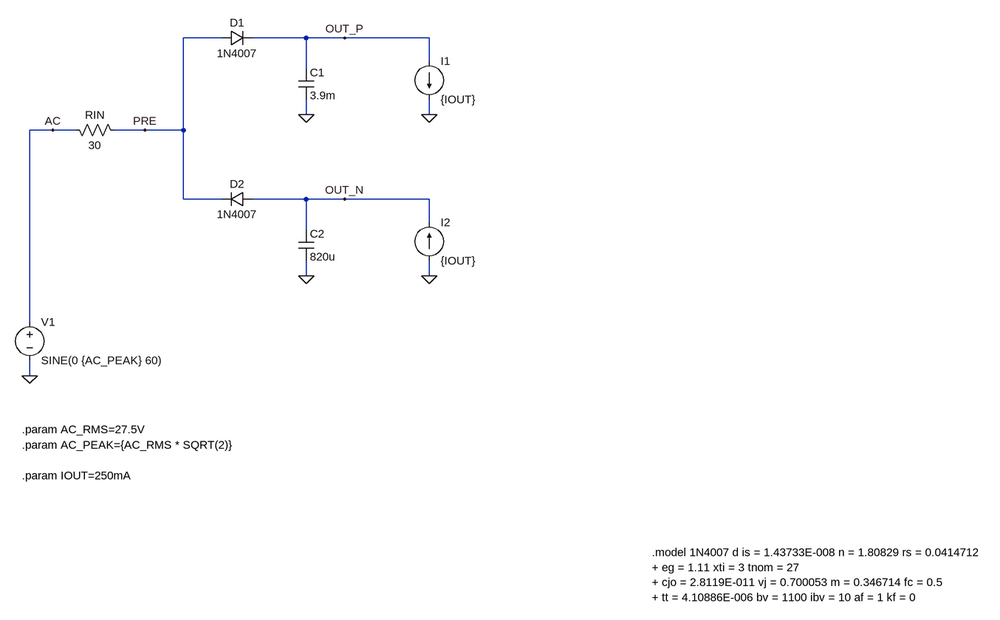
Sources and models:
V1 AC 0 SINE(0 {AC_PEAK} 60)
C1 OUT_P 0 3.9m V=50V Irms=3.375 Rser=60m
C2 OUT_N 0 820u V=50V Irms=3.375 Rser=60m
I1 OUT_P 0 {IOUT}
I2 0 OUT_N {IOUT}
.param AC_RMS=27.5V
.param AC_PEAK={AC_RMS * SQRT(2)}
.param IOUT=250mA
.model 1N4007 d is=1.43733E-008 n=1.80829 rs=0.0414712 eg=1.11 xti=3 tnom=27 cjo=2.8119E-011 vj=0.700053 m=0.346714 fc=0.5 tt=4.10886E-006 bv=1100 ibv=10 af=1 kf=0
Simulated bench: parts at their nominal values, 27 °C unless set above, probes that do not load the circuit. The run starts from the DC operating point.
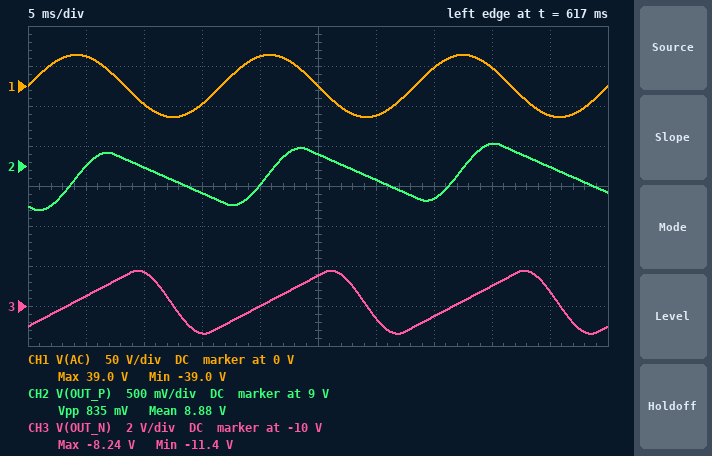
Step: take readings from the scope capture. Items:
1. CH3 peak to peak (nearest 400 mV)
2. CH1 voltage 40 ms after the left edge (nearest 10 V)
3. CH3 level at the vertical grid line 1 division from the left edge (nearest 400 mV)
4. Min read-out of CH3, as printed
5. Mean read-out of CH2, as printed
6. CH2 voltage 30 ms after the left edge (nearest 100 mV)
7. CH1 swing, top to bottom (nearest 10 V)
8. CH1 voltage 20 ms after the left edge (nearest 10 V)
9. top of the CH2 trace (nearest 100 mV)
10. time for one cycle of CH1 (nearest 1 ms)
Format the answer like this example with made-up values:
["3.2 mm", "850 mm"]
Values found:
["3.2 V", "20 V", "-9.6 V", "-11.4 V", "8.88 V", "8.8 V", "80 V", "40 V", "9.3 V", "17 ms"]
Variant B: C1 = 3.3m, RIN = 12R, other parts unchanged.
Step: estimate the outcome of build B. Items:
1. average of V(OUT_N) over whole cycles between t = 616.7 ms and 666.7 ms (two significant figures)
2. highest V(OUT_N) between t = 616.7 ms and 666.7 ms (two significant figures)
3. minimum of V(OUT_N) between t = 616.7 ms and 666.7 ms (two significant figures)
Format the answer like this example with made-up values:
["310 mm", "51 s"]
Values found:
["-22 V", "-21 V", "-24 V"]
